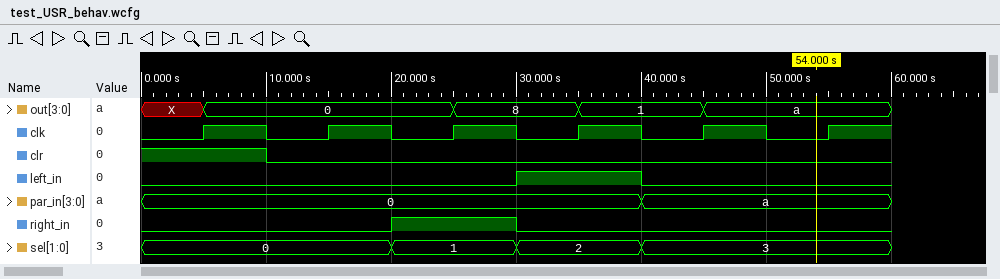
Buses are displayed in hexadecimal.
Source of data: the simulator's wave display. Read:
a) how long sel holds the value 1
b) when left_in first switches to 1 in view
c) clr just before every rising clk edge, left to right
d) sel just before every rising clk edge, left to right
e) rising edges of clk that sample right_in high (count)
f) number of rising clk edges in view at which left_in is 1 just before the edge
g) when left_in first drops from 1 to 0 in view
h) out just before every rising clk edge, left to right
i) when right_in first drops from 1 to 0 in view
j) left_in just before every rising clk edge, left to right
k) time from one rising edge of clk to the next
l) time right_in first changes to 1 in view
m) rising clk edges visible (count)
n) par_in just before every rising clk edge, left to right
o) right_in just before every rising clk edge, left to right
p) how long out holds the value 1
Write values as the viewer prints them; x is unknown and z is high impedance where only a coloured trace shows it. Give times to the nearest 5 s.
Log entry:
10 s
30 s
1 0 0 0 0 0
0, 0, 1, 2, 3, 3
1
1
40 s
X, 0, 0, 8, 1, a
30 s
0 0 0 1 0 0
10 s
20 s
6
0, 0, 0, 0, a, a
0 0 1 0 0 0
10 s
